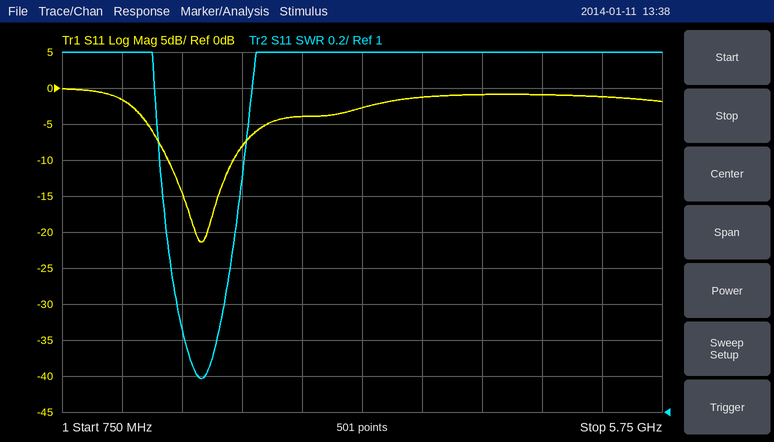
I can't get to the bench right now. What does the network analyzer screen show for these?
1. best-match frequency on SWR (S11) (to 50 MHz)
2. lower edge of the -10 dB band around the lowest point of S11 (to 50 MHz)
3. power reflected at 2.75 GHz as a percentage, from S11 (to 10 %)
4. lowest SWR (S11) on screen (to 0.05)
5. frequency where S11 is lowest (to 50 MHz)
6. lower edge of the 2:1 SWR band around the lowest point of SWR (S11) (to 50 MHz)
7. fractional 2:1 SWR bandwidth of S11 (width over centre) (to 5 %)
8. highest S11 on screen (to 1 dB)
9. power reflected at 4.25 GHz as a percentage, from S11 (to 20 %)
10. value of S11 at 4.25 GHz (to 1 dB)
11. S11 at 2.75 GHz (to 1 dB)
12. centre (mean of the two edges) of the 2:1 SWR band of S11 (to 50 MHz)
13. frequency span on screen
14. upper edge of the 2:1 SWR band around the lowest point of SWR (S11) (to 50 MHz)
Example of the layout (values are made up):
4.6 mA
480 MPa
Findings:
1.90 GHz
1.65 GHz
40 %
1.20
1.90 GHz
1.60 GHz
30 %
0 dB
80 %
-1 dB
-4 dB
1.90 GHz
5 GHz
2.20 GHz
